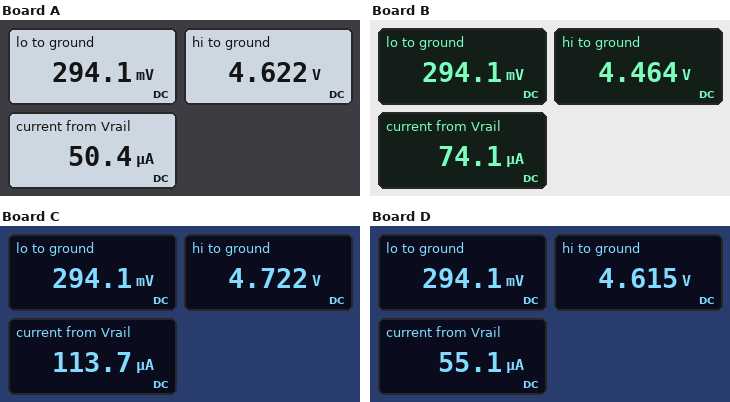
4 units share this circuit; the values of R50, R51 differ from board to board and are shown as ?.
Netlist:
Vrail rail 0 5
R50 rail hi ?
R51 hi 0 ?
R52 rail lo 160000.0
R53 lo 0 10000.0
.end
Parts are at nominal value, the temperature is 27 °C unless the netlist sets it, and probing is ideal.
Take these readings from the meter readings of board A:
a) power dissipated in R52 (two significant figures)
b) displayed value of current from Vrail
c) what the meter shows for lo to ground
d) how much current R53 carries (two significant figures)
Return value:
140 µW
50.4 µA
294.1 mV
29 µA
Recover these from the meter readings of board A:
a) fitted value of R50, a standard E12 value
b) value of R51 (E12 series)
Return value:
18 kΩ
220 kΩ
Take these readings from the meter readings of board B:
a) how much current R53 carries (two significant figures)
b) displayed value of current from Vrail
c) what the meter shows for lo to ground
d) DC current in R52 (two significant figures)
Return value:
29 µA
74.1 µA
294.1 mV
29 µA
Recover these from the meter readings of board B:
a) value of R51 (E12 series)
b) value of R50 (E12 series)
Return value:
100 kΩ
12 kΩ
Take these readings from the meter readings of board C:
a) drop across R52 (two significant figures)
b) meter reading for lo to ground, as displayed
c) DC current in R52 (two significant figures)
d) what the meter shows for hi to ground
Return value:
4.7 V
294.1 mV
29 µA
4.722 V
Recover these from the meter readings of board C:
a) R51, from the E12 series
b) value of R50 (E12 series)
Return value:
56 kΩ
3.3 kΩ
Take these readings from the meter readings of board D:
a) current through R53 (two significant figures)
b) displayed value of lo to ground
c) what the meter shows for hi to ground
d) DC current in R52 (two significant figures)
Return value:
29 µA
294.1 mV
4.615 V
29 µA
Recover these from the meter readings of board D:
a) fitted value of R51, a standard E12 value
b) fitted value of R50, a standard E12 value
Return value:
180 kΩ
15 kΩ
